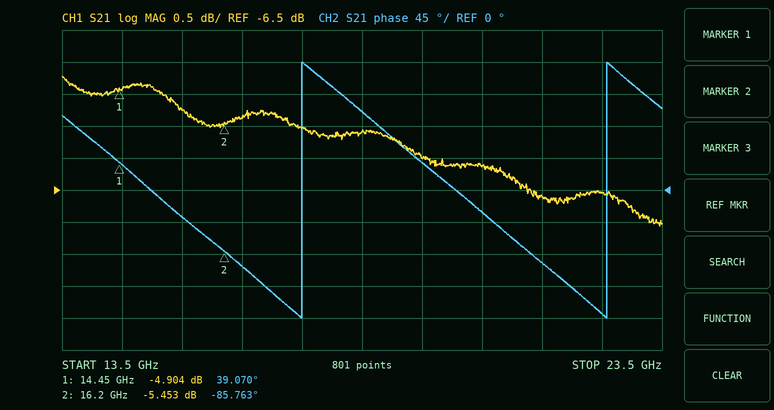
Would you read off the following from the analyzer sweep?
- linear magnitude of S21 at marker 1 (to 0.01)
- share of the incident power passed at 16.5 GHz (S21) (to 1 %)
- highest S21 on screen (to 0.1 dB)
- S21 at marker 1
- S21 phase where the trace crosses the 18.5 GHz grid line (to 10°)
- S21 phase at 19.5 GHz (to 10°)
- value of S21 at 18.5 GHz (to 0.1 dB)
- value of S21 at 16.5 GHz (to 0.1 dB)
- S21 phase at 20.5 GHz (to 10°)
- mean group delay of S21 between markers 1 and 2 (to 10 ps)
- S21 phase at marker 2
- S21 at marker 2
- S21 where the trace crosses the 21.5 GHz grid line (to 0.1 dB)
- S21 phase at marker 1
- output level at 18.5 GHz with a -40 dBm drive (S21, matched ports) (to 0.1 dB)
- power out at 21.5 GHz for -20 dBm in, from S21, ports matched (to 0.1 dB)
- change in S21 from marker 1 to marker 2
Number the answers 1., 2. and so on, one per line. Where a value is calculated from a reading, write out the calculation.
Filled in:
1. 10^(-4.904/20) ≈ 0.57
2. 10^(-5.4/10) ≈ 29 %
3. -4.7 dB
4. -4.904 dB
5. 110°
6. 40°
7. -5.6 dB
8. -5.4 dB
9. -30°
10. −(-85.763° − (39.07°))/(360° × 1.75 GHz) ≈ 198 ps, so 200 ps to the nearest 10 ps
11. -85.763°
12. -5.453 dB
13. -6.6 dB
14. 39.070°
15. -40 dBm + (-5.6 dB) = -45.6 dBm
16. -20 dBm + (-6.6 dB) = -26.6 dBm
17. -5.453 − (-4.904) = -0.549 dB
